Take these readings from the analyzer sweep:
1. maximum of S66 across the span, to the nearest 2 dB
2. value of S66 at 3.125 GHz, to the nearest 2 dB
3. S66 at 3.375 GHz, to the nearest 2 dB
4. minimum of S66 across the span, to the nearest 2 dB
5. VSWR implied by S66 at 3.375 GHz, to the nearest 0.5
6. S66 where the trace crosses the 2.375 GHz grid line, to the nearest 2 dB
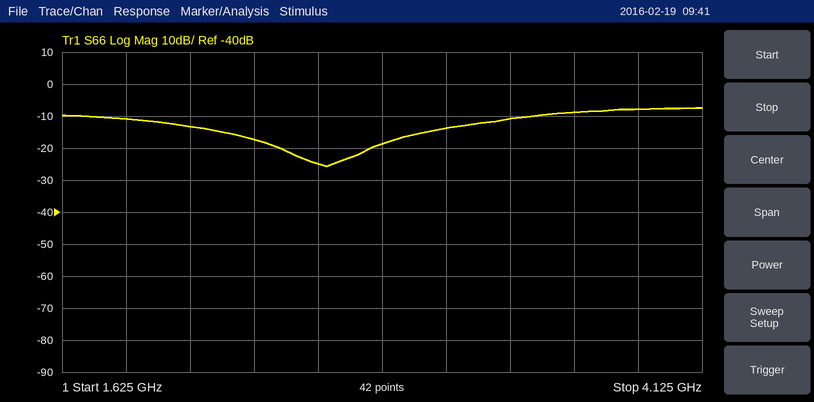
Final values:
-8 dB
-14 dB
-10 dB
-26 dB
2.0
-18 dB
